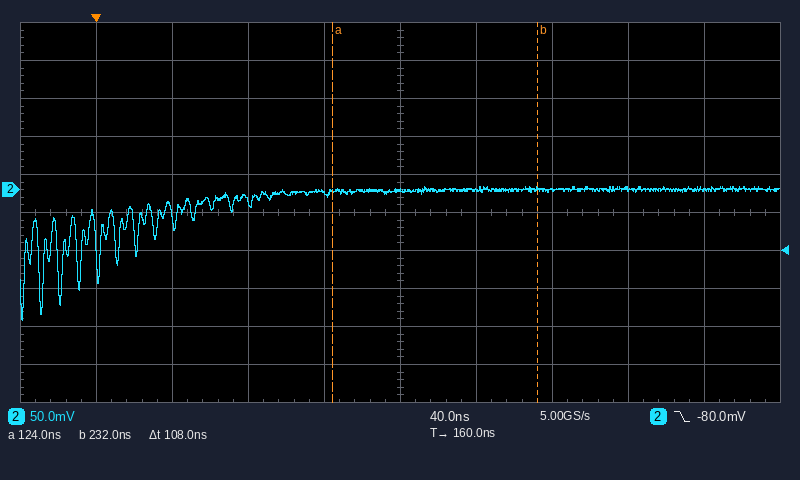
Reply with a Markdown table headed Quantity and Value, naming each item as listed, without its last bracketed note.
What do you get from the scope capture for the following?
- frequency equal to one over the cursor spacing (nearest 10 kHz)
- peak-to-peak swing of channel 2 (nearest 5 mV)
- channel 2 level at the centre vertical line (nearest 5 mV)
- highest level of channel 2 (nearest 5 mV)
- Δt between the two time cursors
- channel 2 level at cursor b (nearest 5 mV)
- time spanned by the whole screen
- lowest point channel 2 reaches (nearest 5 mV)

| Quantity | Value |
|---|---|
| frequency equal to one over the cursor spacing | 9.26 MHz |
| peak-to-peak swing of channel 2 | 175 mV |
| channel 2 level at the centre vertical line | 0 mV |
| highest level of channel 2 | 5 mV |
| Δt between the two time cursors | 108 ns |
| channel 2 level at cursor b | 0 mV |
| time spanned by the whole screen | 400 ns |
| lowest point channel 2 reaches | -170 mV |
